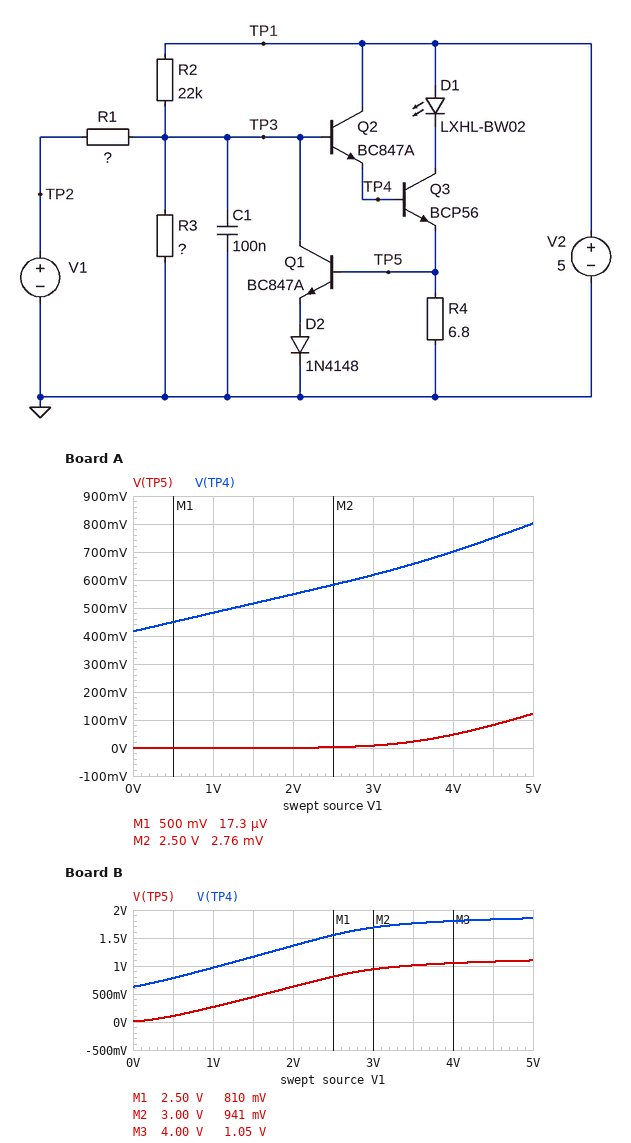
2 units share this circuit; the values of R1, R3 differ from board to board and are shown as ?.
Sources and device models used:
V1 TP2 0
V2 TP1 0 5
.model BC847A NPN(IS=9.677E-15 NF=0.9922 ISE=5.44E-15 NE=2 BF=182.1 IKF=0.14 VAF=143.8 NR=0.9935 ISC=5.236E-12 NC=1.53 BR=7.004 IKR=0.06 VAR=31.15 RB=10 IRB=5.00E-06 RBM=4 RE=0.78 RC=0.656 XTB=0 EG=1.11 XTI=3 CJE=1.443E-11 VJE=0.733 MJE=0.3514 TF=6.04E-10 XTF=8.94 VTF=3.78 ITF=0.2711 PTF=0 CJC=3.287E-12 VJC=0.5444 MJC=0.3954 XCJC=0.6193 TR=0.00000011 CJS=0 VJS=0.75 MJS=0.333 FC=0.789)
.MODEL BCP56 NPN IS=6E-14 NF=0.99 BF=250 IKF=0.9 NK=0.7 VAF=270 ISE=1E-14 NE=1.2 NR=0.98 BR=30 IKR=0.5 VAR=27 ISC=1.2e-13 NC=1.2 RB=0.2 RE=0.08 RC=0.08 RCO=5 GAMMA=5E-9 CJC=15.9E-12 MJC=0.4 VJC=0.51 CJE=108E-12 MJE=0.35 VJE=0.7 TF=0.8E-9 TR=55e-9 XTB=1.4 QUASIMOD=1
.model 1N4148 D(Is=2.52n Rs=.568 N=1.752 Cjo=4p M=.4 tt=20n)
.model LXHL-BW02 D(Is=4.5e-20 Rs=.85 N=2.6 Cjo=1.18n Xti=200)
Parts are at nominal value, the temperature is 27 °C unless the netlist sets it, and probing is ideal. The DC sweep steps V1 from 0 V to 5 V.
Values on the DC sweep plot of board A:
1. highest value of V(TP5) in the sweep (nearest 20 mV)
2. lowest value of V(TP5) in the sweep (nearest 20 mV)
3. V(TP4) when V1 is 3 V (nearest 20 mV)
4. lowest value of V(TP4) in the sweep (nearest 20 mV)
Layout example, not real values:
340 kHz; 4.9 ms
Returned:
120 mV; 0 V; 620 mV; 420 mV
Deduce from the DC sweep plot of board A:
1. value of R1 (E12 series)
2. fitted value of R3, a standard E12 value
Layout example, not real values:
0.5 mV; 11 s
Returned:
27 kΩ; 4.7 kΩ
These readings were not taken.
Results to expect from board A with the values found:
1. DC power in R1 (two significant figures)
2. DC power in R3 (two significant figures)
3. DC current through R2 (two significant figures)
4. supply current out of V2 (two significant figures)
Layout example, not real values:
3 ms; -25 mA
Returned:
22 µW; 130 µW; 190 µA; 190 µA
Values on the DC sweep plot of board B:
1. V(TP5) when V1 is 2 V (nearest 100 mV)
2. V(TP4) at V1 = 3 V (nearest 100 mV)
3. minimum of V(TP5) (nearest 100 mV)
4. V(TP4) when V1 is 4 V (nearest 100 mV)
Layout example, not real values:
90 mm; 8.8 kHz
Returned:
600 mV; 1.7 V; 0 V; 1.8 V
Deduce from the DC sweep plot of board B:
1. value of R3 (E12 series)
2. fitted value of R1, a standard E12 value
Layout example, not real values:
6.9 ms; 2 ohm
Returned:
15 kΩ; 12 kΩ
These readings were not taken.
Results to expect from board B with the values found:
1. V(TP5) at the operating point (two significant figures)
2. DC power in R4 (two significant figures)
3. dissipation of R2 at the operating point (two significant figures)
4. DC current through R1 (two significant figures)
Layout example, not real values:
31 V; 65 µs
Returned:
11 mV; 19 µW; 670 µW; 97 µA
